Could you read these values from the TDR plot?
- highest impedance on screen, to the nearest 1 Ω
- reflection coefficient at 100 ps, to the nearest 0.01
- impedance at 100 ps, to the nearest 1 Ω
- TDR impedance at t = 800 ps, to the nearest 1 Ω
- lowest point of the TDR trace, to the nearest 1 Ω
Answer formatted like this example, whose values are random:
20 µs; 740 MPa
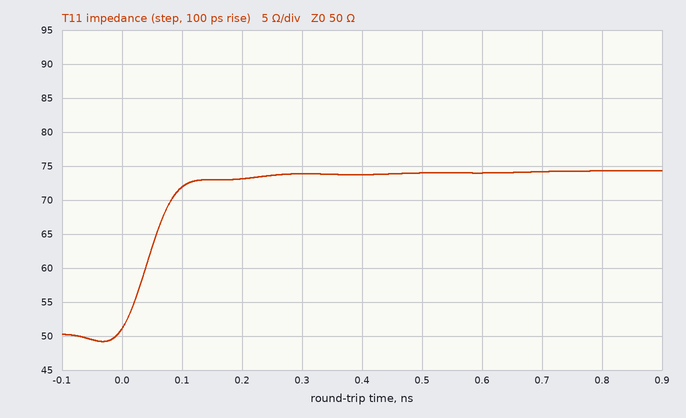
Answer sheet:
74 Ω; +0.18; 72 Ω; 74 Ω; 49 Ω
